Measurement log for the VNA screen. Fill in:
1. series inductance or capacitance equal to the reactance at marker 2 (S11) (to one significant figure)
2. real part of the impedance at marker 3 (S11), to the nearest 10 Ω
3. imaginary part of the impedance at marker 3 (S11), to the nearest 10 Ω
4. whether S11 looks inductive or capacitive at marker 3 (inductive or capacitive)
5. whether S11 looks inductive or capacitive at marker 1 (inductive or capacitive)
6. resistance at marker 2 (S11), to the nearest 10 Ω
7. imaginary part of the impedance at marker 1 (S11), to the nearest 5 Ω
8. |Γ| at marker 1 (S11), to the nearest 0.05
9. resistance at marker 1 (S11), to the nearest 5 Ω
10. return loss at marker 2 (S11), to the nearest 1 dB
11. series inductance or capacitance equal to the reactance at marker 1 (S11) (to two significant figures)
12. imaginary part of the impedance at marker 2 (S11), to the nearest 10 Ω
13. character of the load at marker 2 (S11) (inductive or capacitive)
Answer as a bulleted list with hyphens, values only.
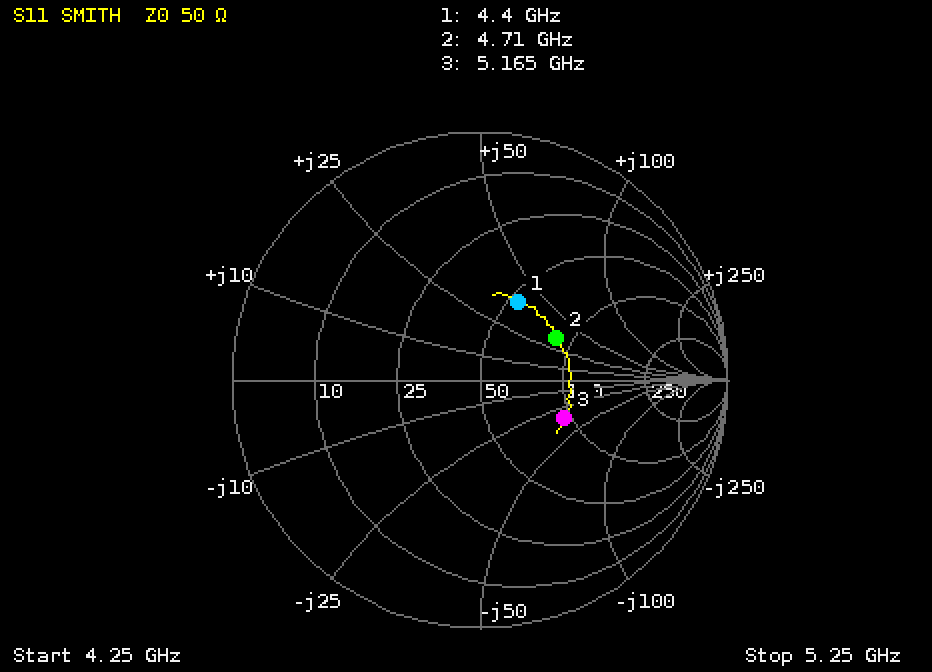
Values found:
- 1 nH
- 90 Ω
- -30 Ω
- capacitive
- inductive
- 90 Ω
- +40 Ω
- 0.35
- 55 Ω
- 9 dB
- 1.4 nH
- +30 Ω
- inductive
